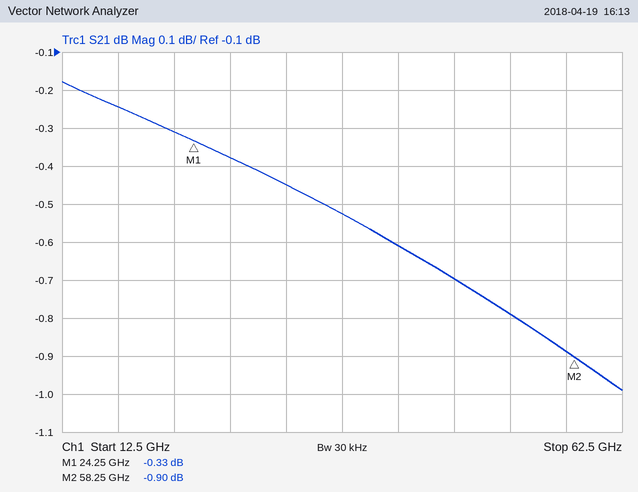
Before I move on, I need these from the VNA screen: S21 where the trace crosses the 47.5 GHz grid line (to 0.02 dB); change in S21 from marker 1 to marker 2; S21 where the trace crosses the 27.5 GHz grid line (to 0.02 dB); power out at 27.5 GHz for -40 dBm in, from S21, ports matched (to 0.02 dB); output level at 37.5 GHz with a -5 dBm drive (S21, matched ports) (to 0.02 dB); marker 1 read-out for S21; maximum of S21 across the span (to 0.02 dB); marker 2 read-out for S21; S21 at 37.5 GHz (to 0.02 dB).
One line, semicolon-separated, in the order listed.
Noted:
-0.70 dB; -0.57 dB; -0.38 dB; -40.38 dBm; -5.52 dBm; -0.33 dB; -0.18 dB; -0.90 dB; -0.52 dB
